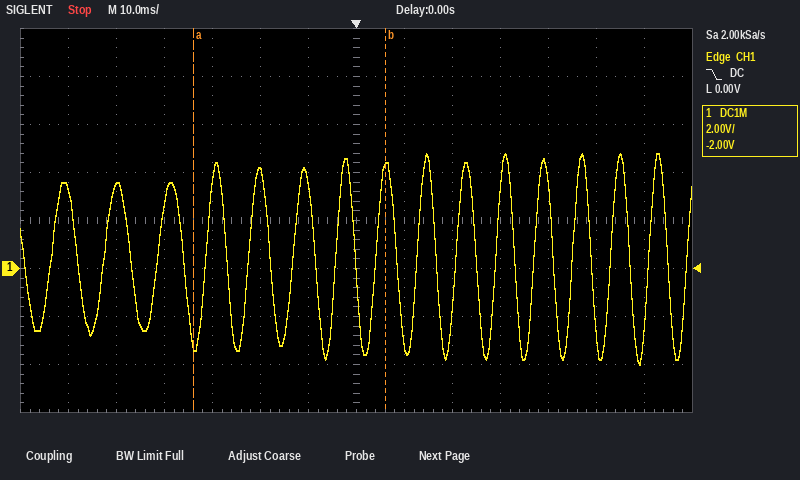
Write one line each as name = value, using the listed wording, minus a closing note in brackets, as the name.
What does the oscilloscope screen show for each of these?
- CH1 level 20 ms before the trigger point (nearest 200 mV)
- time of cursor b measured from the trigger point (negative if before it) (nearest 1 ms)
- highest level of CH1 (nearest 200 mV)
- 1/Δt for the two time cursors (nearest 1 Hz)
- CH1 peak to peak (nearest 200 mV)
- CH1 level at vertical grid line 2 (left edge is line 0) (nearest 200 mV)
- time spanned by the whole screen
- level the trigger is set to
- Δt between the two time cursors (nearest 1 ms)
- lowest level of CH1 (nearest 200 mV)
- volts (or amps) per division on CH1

CH1 level 20 ms before the trigger point = 4.0 V
time of cursor b measured from the trigger point (negative if before it) = +6 ms
highest level of CH1 = 4.8 V
1/Δt for the two time cursors = 25 Hz
CH1 peak to peak = 8.8 V
CH1 level at vertical grid line 2 (left edge is line 0) = 3.4 V
time spanned by the whole screen = 140 ms
level the trigger is set to = 0.00 V
Δt between the two time cursors = 40 ms
lowest level of CH1 = -4.0 V
volts (or amps) per division on CH1 = 2 V
